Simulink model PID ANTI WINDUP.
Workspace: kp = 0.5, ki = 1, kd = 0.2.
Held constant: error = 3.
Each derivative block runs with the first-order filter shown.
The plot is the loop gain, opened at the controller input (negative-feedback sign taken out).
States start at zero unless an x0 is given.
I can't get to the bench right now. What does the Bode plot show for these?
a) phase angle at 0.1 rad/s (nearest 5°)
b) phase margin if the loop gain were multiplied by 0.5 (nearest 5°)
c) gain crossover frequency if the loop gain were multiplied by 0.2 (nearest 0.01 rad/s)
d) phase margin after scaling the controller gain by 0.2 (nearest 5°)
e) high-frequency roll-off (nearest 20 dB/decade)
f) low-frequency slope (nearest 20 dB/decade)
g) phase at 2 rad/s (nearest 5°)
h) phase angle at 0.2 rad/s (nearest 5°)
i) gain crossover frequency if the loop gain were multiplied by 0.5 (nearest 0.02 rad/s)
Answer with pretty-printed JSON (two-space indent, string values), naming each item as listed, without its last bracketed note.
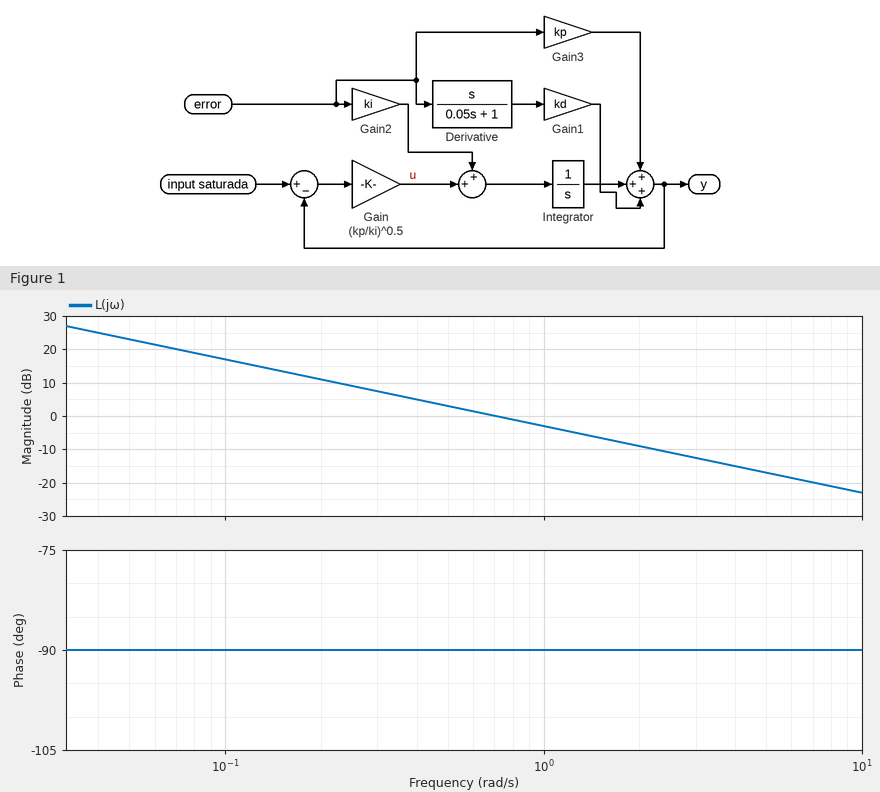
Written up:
{
  "phase angle at 0.1 rad/s": "-90°",
  "phase margin if the loop gain were multiplied by 0.5": "90°",
  "gain crossover frequency if the loop gain were multiplied by 0.2": "0.14 rad/s",
  "phase margin after scaling the controller gain by 0.2": "90°",
  "high-frequency roll-off": "-20 dB/decade",
  "low-frequency slope": "-20 dB/decade",
  "phase at 2 rad/s": "-90°",
  "phase angle at 0.2 rad/s": "-90°",
  "gain crossover frequency if the loop gain were multiplied by 0.5": "0.36 rad/s"
}
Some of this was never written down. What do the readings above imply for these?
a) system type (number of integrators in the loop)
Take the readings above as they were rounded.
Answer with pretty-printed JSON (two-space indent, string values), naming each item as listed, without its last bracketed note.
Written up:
{
  "system type": "1"
}
